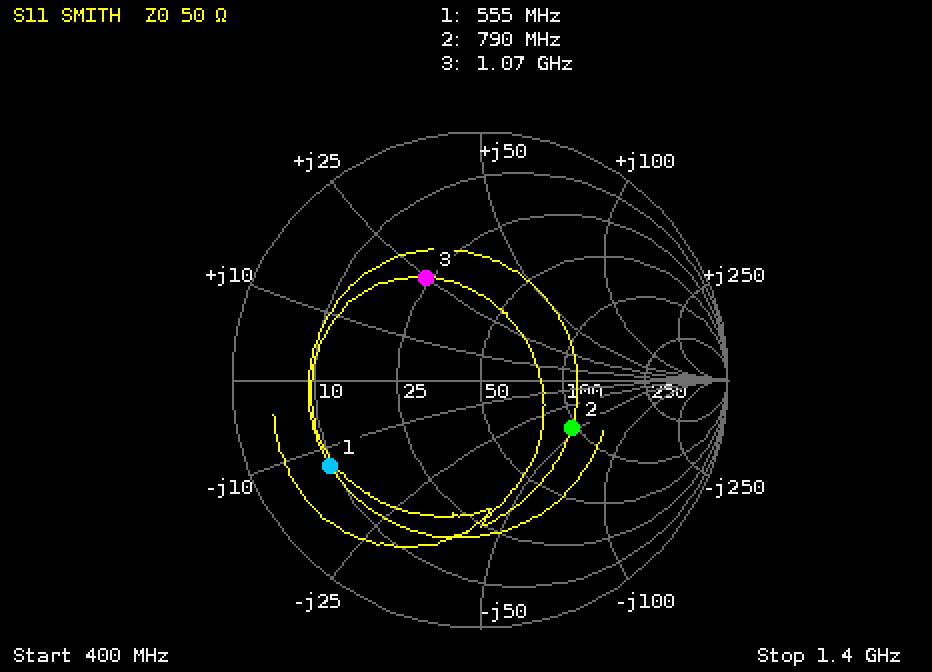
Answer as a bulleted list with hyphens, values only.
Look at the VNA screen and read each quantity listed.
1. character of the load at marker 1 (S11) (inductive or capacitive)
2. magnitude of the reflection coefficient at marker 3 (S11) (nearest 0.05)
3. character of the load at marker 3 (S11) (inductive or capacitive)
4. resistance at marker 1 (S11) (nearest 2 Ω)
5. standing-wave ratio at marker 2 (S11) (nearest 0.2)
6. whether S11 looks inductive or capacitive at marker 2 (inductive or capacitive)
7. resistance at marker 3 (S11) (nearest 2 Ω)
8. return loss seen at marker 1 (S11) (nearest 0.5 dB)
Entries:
- capacitive
- 0.45
- inductive
- 10 Ω
- 2.4
- capacitive
- 24 Ω
- 3.0 dB
